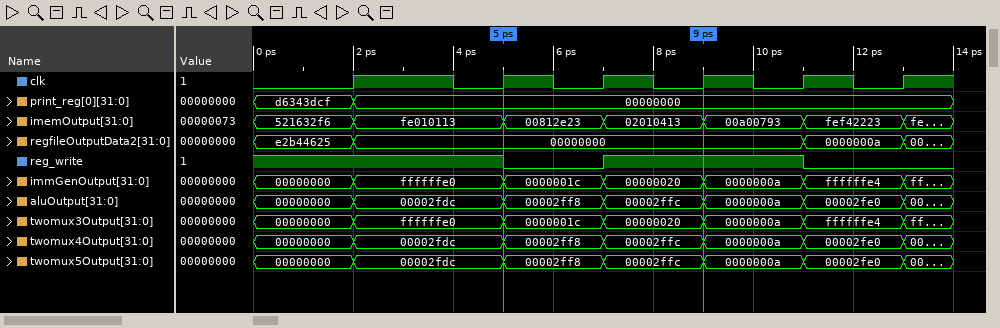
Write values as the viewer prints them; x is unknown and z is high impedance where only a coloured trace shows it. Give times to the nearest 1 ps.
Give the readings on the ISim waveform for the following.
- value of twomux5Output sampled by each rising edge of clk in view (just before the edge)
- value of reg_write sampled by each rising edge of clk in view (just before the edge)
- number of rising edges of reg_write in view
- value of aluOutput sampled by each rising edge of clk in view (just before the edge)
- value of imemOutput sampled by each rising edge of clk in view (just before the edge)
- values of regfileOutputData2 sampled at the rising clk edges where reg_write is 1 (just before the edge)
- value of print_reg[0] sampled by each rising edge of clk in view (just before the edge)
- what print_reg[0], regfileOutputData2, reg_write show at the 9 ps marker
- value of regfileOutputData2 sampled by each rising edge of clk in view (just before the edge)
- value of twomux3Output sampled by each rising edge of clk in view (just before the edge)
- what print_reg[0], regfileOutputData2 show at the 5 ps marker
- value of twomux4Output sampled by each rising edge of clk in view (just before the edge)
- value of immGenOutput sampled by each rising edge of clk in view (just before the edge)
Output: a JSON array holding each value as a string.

["00000000, 00002fdc, 00002ff8, 00002ffc, 0000000a, 00002fe0", "1 1 0 1 1 0", "1", "00000000, 00002fdc, 00002ff8, 00002ffc, 0000000a, 00002fe0", "521632f6, fe010113, 00812e23, 02010413, 00a00793, fef42223", "e2b44625, 00000000, 00000000, 00000000", "d6343dcf, 00000000, 00000000, 00000000, 00000000, 00000000", "print_reg[0]=00000000, regfileOutputData2=00000000, reg_write=1", "e2b44625, 00000000, 00000000, 00000000, 00000000, 0000000a", "00000000, ffffffe0, 0000001c, 00000020, 0000000a, ffffffe4", "print_reg[0]=00000000, regfileOutputData2=00000000", "00000000, 00002fdc, 00002ff8, 00002ffc, 0000000a, 00002fe0", "00000000, ffffffe0, 0000001c, 00000020, 0000000a, ffffffe4"]
